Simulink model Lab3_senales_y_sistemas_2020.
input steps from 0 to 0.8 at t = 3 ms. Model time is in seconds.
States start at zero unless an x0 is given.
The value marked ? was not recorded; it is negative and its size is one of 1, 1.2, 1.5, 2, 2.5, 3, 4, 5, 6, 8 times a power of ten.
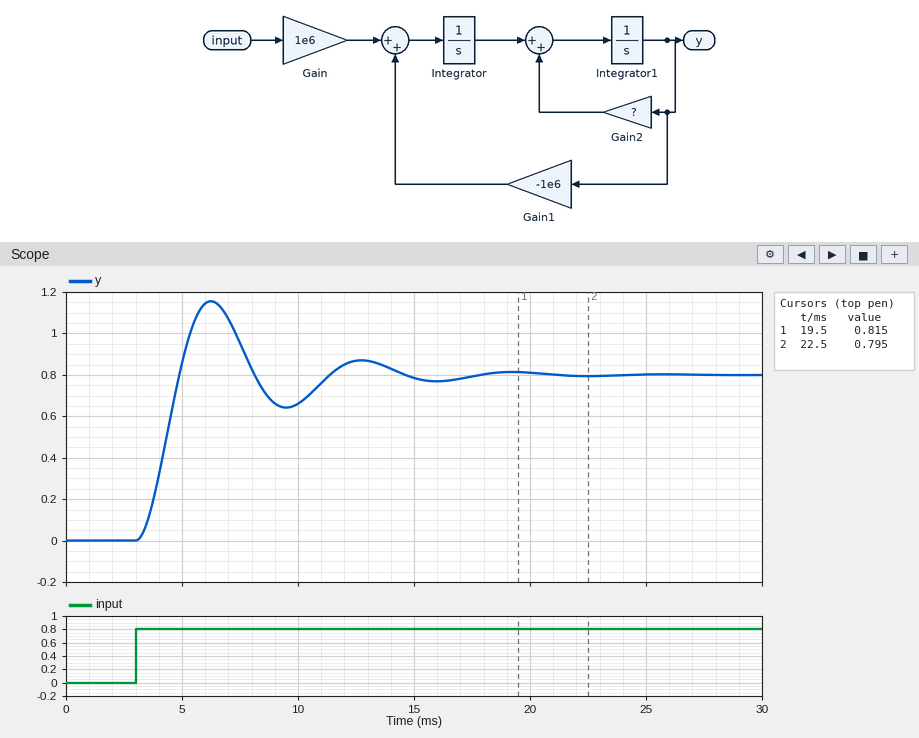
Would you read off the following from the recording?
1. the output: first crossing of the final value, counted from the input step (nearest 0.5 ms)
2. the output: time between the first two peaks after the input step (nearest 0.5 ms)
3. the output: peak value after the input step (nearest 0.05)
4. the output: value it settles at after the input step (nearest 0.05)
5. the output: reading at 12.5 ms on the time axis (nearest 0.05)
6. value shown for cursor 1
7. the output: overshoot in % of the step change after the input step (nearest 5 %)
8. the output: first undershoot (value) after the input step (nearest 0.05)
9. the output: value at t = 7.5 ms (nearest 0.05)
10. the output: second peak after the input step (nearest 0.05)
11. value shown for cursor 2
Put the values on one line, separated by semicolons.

2.0 ms; 6.5 ms; 1.15; 0.80; 0.85; 0.815; 45 %; 0.65; 0.95; 0.85; 0.795
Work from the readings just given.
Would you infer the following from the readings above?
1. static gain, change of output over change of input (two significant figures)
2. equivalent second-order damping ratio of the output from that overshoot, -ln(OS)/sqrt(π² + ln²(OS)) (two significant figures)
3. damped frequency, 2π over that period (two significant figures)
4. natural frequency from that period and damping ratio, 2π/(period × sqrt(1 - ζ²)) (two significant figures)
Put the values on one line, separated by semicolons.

1.0; 0.25; 0.97 rad/ms; 1.00 rad/ms
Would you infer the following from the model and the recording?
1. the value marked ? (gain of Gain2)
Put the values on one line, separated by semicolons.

-500
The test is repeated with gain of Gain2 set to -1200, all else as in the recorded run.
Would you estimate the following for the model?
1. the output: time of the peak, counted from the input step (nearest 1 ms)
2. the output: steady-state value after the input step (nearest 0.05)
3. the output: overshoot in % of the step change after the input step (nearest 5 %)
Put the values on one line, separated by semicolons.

4 ms; 0.80; 10 %
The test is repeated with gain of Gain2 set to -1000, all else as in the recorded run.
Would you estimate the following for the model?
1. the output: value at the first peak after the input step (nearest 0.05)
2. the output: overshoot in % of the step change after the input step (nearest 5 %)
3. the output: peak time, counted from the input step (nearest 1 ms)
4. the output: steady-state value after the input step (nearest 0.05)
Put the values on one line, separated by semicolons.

0.95; 15 %; 4 ms; 0.80
